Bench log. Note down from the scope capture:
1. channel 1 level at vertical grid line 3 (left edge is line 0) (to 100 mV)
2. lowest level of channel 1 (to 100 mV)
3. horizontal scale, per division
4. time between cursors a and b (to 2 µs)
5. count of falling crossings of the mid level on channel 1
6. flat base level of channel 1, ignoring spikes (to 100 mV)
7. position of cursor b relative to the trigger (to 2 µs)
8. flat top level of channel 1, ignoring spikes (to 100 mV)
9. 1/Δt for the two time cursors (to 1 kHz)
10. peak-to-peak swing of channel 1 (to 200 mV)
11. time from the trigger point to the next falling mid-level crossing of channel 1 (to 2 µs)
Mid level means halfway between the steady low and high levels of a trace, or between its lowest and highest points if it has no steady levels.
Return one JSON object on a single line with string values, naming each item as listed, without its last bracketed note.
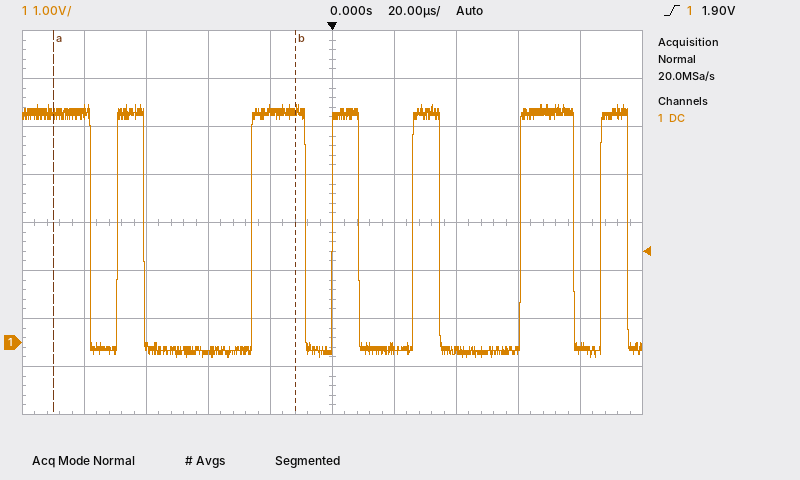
{"channel 1 level at vertical grid line 3 (left edge is line 0)": "-200 mV", "lowest level of channel 1": "-300 mV", "horizontal scale, per division": "20 µs", "time between cursors a and b": "78 µs", "count of falling crossings of the mid level on channel 1": "7", "flat base level of channel 1, ignoring spikes": "-200 mV", "position of cursor b relative to the trigger": "-12 µs", "flat top level of channel 1, ignoring spikes": "4.8 V", "1/Δt for the two time cursors": "13 kHz", "peak-to-peak swing of channel 1": "5.2 V", "time from the trigger point to the next falling mid-level crossing of channel 1": "8 µs"}
